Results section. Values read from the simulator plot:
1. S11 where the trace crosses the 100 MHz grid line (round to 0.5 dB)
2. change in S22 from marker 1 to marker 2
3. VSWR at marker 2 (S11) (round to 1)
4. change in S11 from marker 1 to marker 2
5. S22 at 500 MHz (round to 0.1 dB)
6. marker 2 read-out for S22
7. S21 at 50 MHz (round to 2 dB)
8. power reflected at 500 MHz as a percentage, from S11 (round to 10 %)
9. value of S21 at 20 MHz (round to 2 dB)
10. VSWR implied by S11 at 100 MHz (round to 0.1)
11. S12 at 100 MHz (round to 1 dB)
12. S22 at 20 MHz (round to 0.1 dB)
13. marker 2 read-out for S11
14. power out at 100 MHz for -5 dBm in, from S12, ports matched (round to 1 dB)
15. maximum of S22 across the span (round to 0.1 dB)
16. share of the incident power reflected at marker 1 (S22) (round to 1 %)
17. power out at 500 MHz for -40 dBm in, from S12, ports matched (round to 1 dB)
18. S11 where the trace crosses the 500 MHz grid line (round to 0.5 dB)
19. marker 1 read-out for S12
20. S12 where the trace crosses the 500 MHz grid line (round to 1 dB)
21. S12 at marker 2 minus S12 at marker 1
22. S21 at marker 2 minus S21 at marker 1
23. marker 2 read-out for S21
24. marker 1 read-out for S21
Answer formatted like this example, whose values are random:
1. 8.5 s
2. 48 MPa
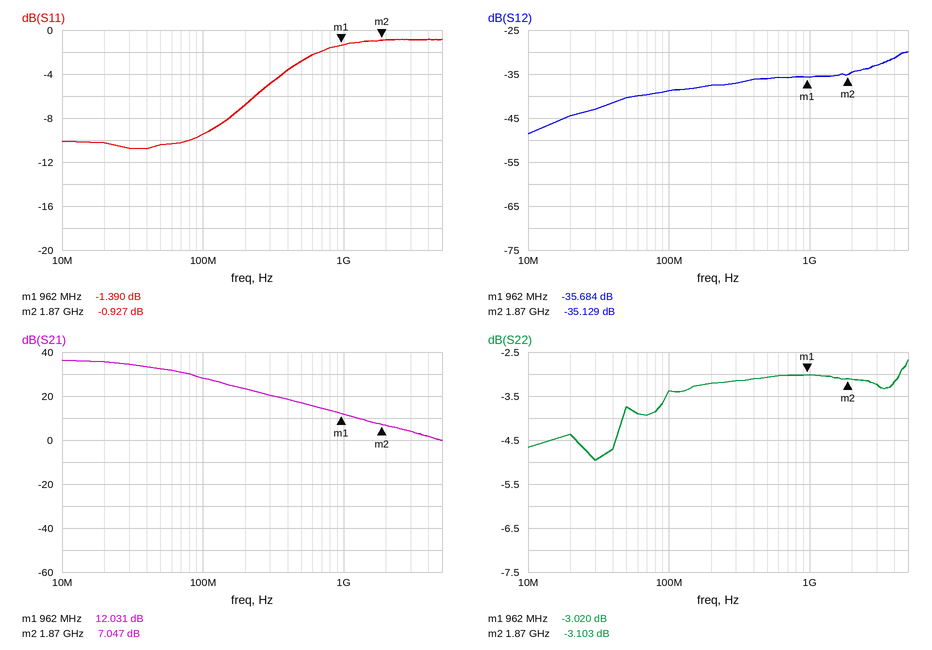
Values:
1. -9.5 dB
2. -0.083 dB
3. 19
4. 0.463 dB
5. -3.1 dB
6. -3.103 dB
7. 32 dB
8. 50 %
9. 36 dB
10. 2.0
11. -39 dB
12. -4.4 dB
13. -0.927 dB
14. -44 dBm
15. -2.7 dB
16. 50 %
17. -76 dBm
18. -3.0 dB
19. -35.684 dB
20. -36 dB
21. 0.555 dB
22. -4.984 dB
23. 7.047 dB
24. 12.031 dB
